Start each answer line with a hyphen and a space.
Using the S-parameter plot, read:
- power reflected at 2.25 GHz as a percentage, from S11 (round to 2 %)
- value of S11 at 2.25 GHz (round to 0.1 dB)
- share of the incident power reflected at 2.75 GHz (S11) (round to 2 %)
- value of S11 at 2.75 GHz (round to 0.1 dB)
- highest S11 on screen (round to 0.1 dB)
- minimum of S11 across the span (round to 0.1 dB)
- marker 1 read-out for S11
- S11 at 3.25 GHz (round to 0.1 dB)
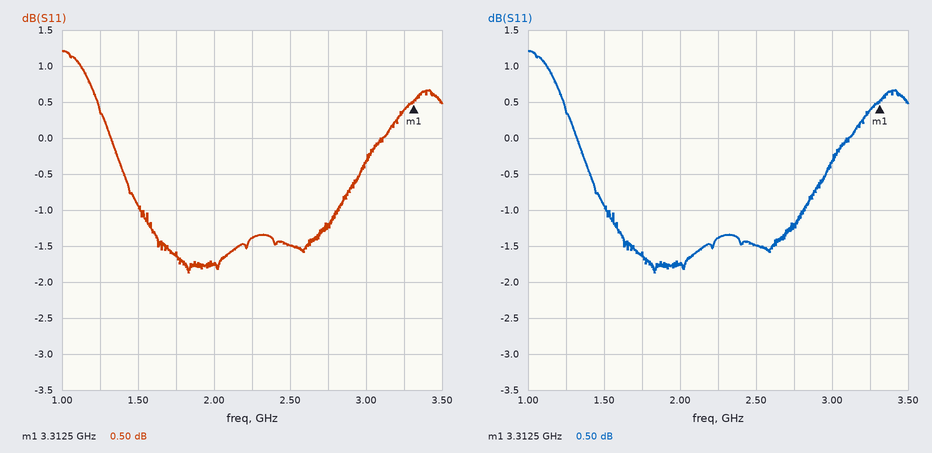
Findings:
- 72 %
- -1.4 dB
- 76 %
- -1.2 dB
- 1.2 dB
- -1.9 dB
- 0.50 dB
- 0.4 dB
